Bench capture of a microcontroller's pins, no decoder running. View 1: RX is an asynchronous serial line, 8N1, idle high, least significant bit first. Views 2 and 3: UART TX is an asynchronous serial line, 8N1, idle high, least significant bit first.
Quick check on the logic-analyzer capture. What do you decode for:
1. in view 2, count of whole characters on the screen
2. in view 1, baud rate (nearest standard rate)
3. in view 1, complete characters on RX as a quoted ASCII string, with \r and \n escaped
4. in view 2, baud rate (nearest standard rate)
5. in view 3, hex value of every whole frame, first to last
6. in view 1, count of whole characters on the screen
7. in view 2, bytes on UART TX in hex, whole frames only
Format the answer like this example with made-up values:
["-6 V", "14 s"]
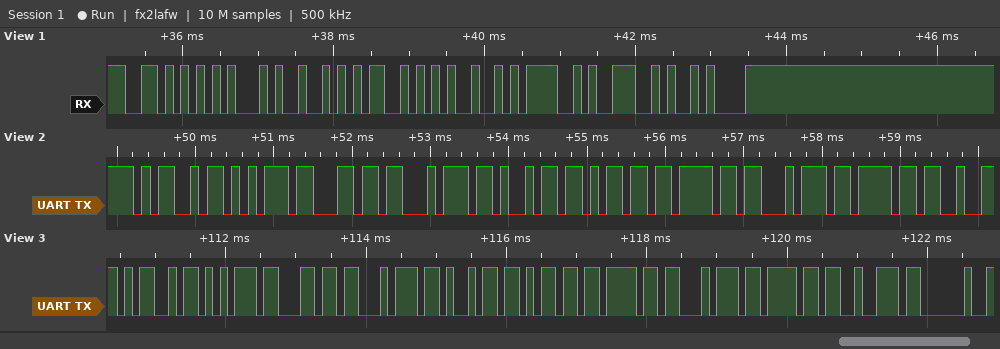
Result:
["9", "9600 baud", "\"VERSION\\n\"", "9600 baud", "4D 75 6C 74 69 6D 6F 74 6F 72 20", "8", "4D 75 6C 74 69 6D 6F 74 6F"]
